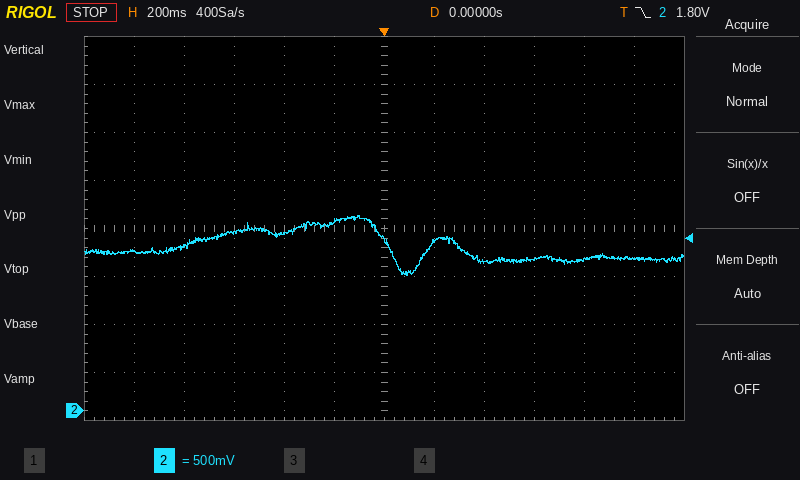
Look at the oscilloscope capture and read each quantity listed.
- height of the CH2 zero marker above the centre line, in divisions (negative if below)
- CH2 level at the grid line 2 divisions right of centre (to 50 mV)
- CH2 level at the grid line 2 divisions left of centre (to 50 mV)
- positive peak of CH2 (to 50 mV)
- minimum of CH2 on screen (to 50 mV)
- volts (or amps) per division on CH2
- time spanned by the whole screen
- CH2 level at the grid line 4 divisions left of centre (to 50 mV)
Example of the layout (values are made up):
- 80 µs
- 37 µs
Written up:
- -3.8 div
- 1.55 V
- 1.85 V
- 2.05 V
- 1.40 V
- 500 mV
- 2.4 s
- 1.70 V
